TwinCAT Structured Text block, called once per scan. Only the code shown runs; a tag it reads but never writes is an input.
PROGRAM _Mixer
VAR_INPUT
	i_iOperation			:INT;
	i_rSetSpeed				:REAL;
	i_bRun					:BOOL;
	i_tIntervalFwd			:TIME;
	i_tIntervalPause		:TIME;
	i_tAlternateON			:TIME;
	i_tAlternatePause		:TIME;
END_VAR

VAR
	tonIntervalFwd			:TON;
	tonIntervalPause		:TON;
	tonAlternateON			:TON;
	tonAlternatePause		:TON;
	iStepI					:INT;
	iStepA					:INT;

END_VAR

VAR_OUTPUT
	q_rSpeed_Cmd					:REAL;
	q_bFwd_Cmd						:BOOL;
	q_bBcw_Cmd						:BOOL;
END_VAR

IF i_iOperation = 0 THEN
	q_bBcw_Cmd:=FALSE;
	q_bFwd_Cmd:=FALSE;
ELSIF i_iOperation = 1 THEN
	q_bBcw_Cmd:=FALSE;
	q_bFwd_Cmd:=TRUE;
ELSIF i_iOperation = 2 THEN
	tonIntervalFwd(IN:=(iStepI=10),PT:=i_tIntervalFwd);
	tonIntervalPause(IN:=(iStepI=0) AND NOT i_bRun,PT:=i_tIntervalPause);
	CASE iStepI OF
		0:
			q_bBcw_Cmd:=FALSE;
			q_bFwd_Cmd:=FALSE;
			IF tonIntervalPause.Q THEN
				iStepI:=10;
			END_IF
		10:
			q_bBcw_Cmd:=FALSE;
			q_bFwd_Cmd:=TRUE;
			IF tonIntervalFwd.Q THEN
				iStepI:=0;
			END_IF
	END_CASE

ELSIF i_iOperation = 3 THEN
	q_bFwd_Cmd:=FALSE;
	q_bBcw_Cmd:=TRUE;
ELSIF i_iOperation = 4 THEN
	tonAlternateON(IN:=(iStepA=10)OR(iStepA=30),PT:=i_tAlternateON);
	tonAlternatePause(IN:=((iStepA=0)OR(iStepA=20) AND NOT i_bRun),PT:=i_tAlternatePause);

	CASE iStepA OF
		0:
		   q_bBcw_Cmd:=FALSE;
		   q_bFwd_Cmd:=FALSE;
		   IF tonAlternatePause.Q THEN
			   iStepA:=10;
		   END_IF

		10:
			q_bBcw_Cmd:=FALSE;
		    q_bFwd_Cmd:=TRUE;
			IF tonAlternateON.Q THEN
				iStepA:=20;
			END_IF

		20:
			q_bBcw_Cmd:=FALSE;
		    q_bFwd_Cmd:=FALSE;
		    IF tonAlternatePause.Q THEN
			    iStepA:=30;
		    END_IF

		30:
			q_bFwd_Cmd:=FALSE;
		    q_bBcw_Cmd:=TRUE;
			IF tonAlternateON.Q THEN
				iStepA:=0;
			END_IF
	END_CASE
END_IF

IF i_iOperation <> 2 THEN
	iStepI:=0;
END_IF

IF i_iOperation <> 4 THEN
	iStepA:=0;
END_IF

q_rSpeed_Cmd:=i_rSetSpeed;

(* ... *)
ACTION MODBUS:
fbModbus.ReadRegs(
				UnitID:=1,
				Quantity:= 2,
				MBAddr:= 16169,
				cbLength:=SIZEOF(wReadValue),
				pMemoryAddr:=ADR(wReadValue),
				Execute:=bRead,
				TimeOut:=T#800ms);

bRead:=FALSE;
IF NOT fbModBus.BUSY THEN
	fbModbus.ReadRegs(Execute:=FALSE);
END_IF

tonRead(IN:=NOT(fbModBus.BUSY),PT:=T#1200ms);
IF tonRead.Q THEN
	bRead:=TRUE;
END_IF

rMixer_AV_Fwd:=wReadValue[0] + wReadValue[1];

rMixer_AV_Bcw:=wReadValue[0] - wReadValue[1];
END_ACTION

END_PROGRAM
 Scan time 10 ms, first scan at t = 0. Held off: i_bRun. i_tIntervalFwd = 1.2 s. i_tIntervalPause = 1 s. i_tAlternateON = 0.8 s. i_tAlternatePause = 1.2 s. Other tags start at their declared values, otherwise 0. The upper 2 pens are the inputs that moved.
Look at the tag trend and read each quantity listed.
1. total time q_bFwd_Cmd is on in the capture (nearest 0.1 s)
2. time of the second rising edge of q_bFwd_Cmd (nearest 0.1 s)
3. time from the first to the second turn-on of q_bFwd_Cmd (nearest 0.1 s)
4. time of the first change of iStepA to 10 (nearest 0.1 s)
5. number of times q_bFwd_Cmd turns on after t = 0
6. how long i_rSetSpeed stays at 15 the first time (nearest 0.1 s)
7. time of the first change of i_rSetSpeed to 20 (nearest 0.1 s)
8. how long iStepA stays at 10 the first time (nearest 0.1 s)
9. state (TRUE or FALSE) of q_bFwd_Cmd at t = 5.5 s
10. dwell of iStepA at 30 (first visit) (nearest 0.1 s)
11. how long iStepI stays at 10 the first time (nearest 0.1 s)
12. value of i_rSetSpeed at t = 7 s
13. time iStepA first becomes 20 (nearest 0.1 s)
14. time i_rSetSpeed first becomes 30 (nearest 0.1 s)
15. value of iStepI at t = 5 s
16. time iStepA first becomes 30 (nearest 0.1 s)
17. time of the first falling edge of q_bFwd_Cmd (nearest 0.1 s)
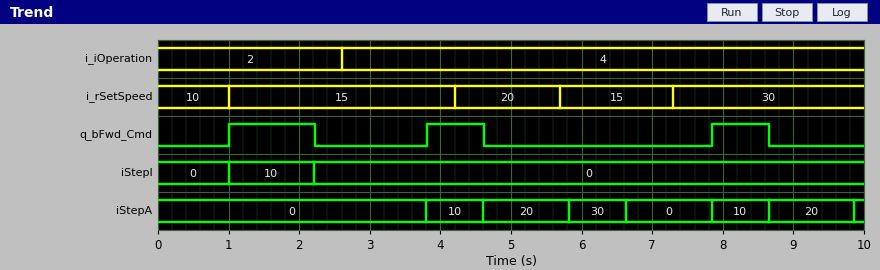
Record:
2.8 s
3.8 s
2.8 s
3.8 s
3
3.2 s
4.2 s
0.8 s
FALSE
0.8 s
1.2 s
15
4.6 s
7.3 s
0
5.8 s
2.2 s
